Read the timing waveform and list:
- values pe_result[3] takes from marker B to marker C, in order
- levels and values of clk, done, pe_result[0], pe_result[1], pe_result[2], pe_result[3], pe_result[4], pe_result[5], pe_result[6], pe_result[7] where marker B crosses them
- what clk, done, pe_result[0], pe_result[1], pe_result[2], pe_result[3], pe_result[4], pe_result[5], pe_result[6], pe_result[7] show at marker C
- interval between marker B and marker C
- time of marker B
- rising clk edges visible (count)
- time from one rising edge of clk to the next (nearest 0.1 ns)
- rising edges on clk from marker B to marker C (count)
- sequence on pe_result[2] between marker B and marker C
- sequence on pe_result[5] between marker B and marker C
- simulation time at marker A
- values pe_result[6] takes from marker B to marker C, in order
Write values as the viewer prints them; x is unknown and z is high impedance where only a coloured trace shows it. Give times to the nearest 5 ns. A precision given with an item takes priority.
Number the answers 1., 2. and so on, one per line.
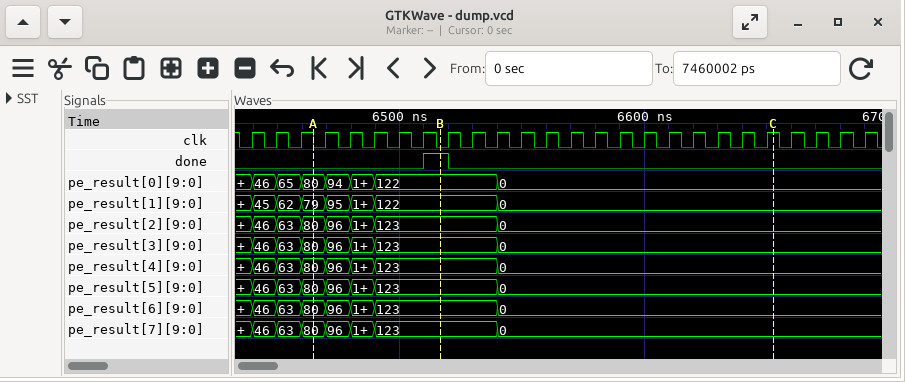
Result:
1. 123, 0
2. clk=0, done=1, pe_result[0]=122, pe_result[1]=122, pe_result[2]=123, pe_result[3]=123, pe_result[4]=123, pe_result[5]=123, pe_result[6]=123, pe_result[7]=123
3. clk=1, done=0, pe_result[0]=0, pe_result[1]=0, pe_result[2]=0, pe_result[3]=0, pe_result[4]=0, pe_result[5]=0, pe_result[6]=0, pe_result[7]=0
4. 135 ns
5. 6515 ns
6. 26
7. 10 ns
8. 14
9. 123, 0
10. 123, 0
11. 6465 ns
12. 123, 0
